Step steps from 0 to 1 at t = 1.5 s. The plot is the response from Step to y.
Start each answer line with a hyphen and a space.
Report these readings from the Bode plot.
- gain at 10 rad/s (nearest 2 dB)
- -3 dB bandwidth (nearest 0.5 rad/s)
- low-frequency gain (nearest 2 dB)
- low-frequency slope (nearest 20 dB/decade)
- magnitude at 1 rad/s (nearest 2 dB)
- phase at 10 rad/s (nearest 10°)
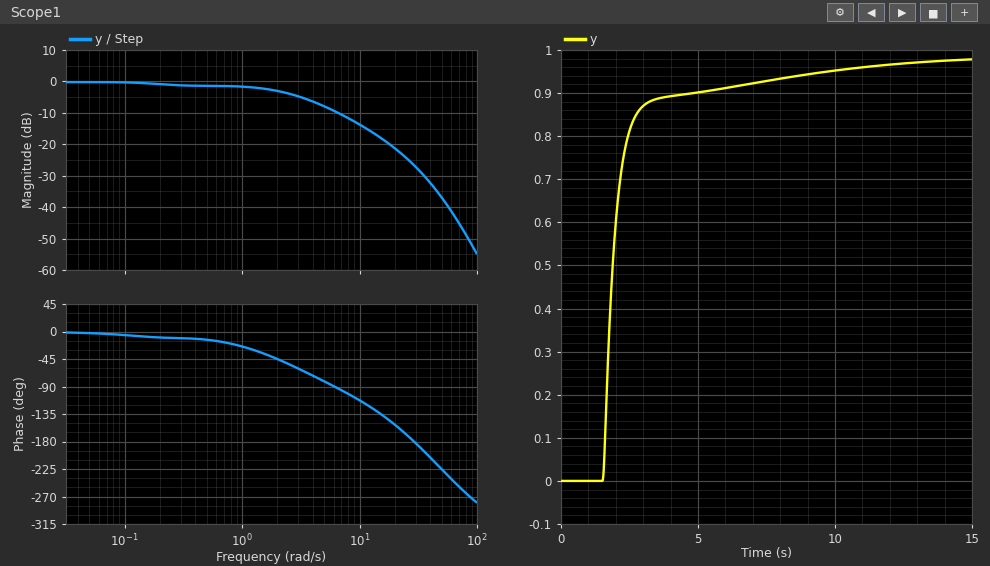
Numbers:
- -14 dB
- 2.0 rad/s
- 0 dB
- 0 dB/decade
- -2 dB
- -110°
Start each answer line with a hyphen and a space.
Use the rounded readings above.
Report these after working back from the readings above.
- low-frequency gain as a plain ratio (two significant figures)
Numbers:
- 1.0
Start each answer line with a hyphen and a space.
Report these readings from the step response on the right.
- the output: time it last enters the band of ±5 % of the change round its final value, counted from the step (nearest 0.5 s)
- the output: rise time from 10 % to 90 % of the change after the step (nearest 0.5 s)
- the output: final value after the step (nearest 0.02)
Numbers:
- 6.0 s
- 1.5 s
- 0.98
